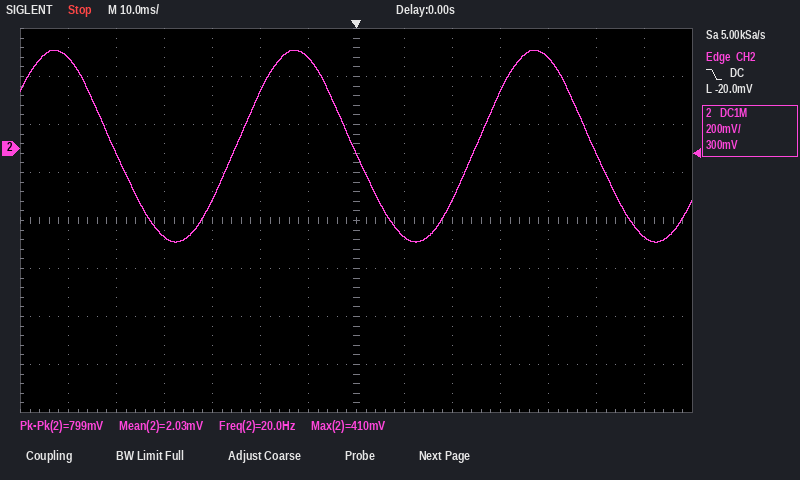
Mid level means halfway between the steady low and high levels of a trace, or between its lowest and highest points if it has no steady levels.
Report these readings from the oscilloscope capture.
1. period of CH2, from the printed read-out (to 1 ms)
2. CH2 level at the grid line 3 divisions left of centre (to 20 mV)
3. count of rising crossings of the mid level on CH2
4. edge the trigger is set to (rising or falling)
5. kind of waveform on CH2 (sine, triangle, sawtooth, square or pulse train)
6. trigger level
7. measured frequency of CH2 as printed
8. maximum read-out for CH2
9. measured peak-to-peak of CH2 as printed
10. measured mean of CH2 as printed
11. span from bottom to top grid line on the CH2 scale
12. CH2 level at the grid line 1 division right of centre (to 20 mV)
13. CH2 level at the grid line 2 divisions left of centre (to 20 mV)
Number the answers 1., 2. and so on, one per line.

1. 50 ms
2. -220 mV
3. 2
4. falling
5. sine
6. -20.0 mV
7. 20.0 Hz
8. 410 mV
9. 799 mV
10. 2.03 mV
11. 1.6 V
12. -360 mV
13. 240 mV
